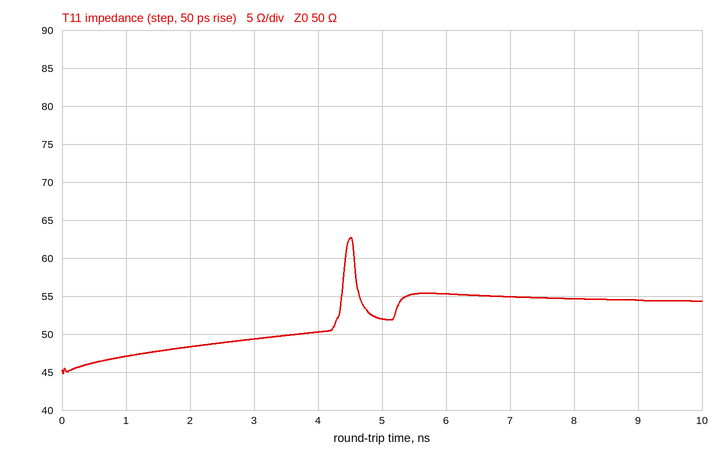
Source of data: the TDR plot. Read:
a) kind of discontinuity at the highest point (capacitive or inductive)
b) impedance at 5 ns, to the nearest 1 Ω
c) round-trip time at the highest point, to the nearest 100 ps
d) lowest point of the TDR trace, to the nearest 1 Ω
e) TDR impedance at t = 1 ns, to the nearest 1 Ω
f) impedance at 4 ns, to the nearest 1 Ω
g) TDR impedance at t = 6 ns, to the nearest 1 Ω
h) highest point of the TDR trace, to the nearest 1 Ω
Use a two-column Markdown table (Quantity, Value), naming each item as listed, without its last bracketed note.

| Quantity | Value |
|---|---|
| kind of discontinuity at the highest point | inductive |
| impedance at 5 ns, to the nearest 1 Ω | 52 Ω |
| round-trip time at the highest point, to the nearest 100 ps | 4.5 ns |
| lowest point of the TDR trace, to the nearest 1 Ω | 45 Ω |
| TDR impedance at t = 1 ns, to the nearest 1 Ω | 47 Ω |
| impedance at 4 ns, to the nearest 1 Ω | 50 Ω |
| TDR impedance at t = 6 ns, to the nearest 1 Ω | 55 Ω |
| highest point of the TDR trace, to the nearest 1 Ω | 63 Ω |
